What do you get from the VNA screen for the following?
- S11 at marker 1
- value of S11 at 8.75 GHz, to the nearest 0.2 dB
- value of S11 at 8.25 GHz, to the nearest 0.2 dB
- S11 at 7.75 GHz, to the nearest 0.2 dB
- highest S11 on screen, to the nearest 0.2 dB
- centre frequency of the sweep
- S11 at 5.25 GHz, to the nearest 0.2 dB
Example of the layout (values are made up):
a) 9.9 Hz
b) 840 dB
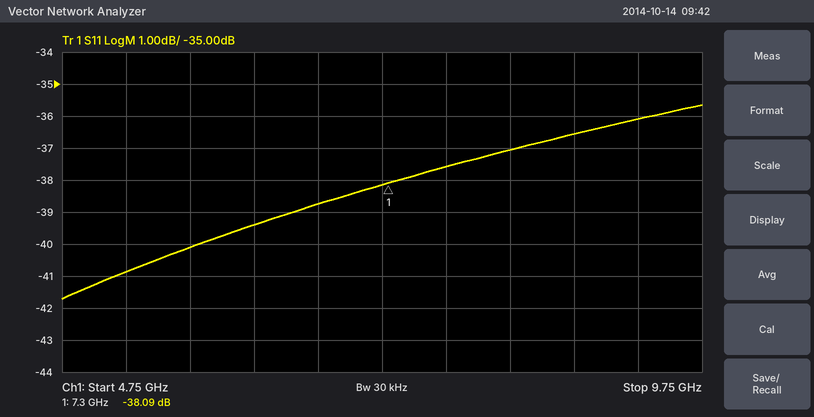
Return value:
a) -38.09 dB
b) -36.6 dB
c) -37.0 dB
d) -37.6 dB
e) -35.6 dB
f) 7.25 GHz
g) -40.8 dB
